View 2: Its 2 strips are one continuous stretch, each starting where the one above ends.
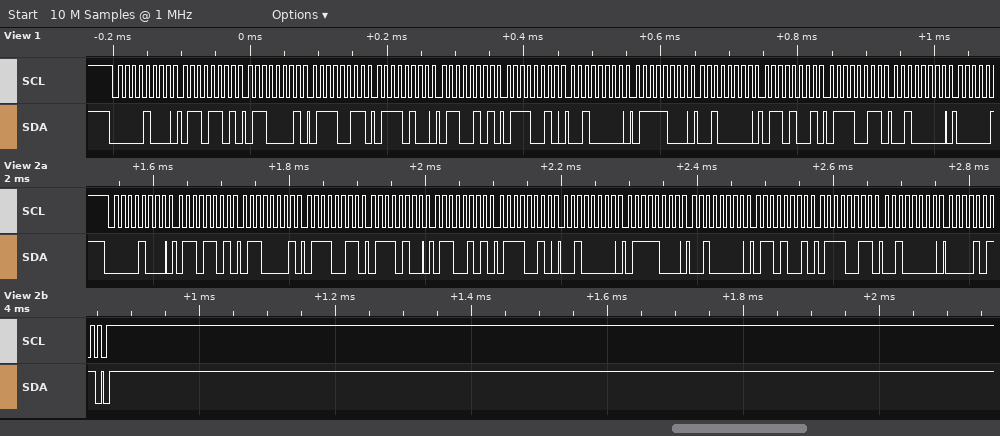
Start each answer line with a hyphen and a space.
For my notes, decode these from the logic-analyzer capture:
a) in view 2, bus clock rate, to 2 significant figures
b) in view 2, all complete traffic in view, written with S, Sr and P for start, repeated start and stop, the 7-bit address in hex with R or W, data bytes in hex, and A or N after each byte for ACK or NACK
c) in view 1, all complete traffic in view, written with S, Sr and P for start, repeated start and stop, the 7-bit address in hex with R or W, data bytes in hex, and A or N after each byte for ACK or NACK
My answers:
- 100 kHz
- S 04W A 6D A 61 A 73 A 74 A 65 A 72 A 20 A 78 A 20 A 69 A 73 A 20 A 0B A P
- S 04W A 6D A 61 A 73 A 74 A 65 A 72 A 20 A 78 A 20 A 69 A 73 A 20 A
